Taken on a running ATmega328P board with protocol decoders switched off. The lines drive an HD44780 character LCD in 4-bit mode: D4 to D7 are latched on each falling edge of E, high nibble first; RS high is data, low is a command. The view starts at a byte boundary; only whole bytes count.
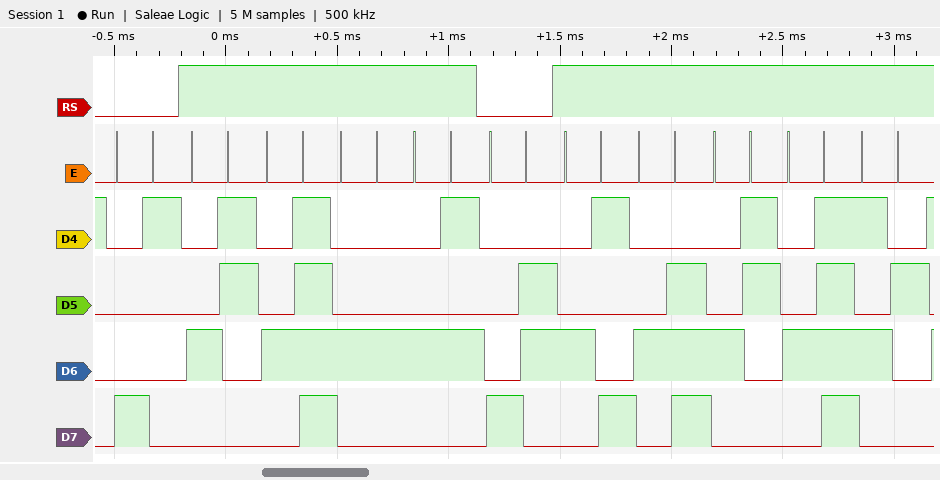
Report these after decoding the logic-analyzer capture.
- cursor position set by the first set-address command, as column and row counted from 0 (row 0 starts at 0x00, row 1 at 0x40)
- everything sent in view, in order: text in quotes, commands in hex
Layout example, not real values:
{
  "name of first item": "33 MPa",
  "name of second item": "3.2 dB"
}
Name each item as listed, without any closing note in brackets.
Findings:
{
  "cursor position set by the first set-address command, as column and row counted from 0": "column 1, row 0",
  "everything sent in view, in order: text in quotes, commands in hex": "0x81 \"CODE\" 0x86 \"INCOR\""
}
